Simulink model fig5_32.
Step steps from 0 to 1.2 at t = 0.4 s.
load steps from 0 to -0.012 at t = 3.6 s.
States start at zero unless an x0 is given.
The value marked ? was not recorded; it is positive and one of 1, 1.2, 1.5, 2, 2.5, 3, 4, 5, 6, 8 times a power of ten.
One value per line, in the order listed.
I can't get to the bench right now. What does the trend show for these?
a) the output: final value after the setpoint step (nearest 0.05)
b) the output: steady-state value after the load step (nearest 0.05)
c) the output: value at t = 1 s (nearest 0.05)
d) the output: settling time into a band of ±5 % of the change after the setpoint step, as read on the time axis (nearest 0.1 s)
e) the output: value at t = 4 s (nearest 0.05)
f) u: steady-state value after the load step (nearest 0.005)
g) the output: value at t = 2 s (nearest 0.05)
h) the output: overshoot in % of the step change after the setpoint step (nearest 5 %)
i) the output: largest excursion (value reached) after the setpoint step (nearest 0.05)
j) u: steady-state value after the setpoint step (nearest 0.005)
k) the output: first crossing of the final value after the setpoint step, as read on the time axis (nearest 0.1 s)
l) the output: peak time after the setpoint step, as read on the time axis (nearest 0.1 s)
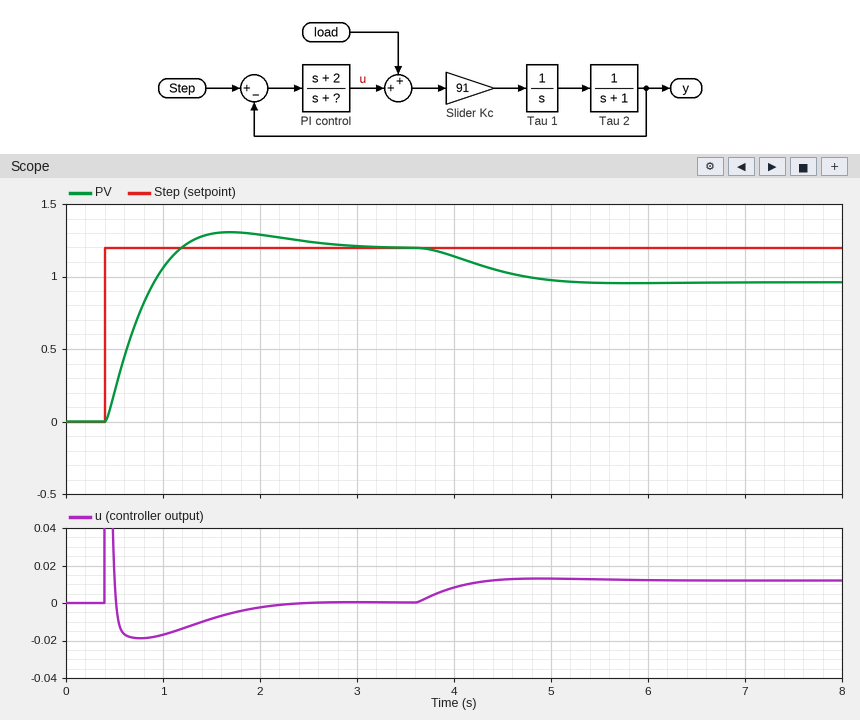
1.20
0.95
1.05
2.3 s
1.15
0.010
1.30
10 %
1.30
0.000
1.2 s
1.7 s
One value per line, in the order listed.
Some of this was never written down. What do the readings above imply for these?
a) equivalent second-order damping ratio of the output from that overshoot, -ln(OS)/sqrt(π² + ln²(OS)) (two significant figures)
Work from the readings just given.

0.59
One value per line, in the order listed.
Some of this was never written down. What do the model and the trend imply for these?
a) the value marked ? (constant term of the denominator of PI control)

40
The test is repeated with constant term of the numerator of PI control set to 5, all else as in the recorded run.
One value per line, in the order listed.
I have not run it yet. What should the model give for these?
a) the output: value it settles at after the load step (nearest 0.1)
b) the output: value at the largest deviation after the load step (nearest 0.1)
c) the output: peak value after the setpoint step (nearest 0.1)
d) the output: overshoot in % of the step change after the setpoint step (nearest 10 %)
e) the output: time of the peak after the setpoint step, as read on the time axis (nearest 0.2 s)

1.1
1.1
1.5
30 %
1.2 s
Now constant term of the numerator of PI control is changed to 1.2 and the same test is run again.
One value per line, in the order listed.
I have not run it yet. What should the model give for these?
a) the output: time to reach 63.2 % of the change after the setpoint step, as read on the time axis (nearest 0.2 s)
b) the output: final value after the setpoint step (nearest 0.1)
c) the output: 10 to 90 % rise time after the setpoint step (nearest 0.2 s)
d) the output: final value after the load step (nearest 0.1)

0.8 s
1.2
0.8 s
0.8
